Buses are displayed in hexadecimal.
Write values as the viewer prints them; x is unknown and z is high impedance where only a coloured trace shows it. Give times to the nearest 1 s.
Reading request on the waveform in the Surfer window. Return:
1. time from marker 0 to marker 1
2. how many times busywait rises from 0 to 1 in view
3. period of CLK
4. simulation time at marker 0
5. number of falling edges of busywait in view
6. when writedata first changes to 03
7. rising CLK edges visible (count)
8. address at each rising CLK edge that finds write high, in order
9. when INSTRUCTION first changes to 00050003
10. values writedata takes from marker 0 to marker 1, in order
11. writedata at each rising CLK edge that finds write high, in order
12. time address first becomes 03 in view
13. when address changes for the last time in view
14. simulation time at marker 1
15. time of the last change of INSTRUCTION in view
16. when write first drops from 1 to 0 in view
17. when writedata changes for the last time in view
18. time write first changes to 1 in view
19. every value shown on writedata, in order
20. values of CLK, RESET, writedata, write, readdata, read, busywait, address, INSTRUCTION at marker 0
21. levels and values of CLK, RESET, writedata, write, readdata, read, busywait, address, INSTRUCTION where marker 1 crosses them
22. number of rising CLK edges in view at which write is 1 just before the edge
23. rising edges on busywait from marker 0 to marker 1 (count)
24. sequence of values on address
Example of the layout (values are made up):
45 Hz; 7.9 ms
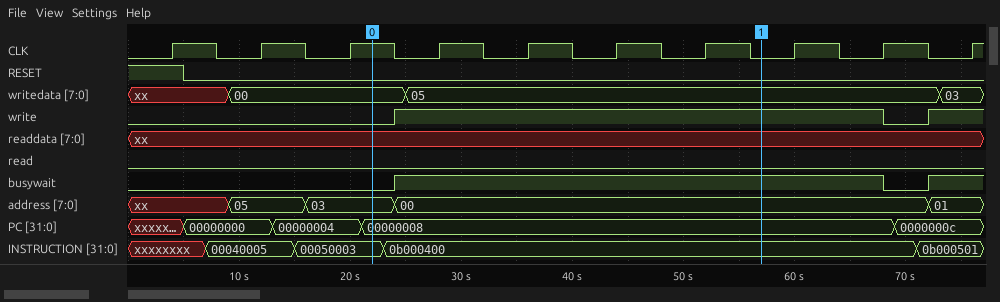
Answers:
35 s; 2; 8 s; 22 s; 1; 73 s; 10; 00, 00, 00, 00, 00, 00, 01; 15 s; 00, 05; 05, 05, 05, 05, 05, 05, 03; 16 s; 72 s; 57 s; 71 s; 68 s; 73 s; 24 s; xx, 00, 05, 03; CLK=1, RESET=0, writedata=00, write=0, readdata=xx, read=0, busywait=0, address=03, INSTRUCTION=00050003; CLK=0, RESET=0, writedata=05, write=1, readdata=xx, read=0, busywait=1, address=00, INSTRUCTION=0b000400; 7; 1; xx, 05, 03, 00, 01
